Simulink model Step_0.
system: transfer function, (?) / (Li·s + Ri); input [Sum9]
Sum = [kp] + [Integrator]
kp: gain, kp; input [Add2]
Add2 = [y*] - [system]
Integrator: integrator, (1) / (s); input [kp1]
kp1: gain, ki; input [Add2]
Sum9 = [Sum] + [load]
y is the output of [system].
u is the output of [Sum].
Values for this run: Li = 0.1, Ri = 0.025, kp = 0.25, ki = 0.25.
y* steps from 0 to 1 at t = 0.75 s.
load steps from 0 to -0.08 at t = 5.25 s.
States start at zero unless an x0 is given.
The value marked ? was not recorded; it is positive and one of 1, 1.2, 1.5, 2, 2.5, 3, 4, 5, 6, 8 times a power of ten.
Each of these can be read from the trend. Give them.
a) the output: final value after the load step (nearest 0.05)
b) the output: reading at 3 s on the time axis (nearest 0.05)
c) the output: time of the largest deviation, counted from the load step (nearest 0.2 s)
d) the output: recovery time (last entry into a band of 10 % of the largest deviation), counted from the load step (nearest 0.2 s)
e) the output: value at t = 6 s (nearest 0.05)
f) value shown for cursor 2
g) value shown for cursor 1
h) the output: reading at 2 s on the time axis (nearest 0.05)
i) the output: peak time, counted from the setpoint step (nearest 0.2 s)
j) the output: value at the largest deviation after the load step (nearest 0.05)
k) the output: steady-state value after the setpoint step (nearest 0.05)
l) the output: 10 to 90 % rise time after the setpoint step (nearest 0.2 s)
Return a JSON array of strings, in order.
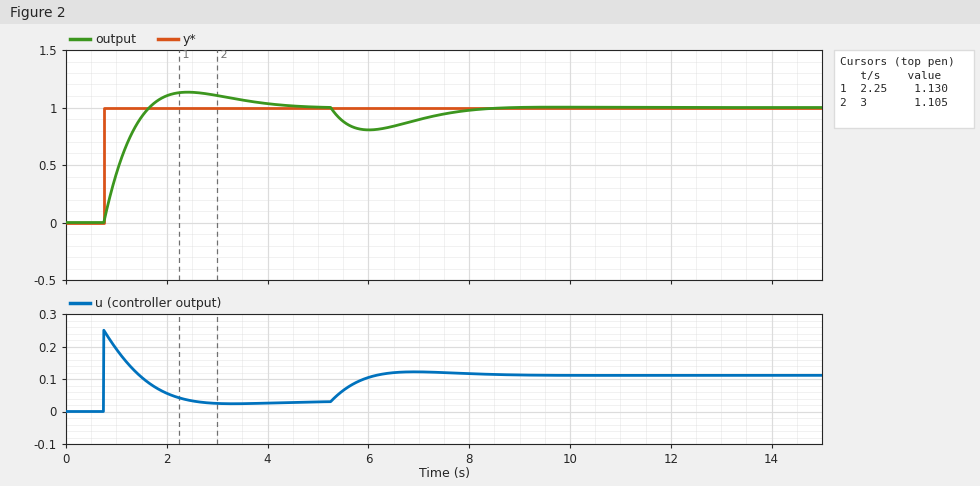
["1.00", "1.10", "0.8 s", "2.8 s", "0.80", "1.105", "1.130", "1.10", "1.6 s", "0.80", "1.00", "0.6 s"]
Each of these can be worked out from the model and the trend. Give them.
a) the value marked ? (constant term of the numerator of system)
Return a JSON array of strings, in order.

["0.8"]
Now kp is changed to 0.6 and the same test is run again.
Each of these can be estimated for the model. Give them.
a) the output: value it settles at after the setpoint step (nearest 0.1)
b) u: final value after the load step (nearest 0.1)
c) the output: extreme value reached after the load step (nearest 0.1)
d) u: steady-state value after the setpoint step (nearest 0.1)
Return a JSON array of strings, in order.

["1.0", "0.1", "0.9", "0.0"]
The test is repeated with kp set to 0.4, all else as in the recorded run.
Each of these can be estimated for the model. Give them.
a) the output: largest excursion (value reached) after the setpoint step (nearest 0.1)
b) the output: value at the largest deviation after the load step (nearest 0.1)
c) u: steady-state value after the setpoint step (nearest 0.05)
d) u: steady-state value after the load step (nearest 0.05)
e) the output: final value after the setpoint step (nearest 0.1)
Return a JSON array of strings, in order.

["1.1", "0.9", "0.05", "0.10", "1.0"]
